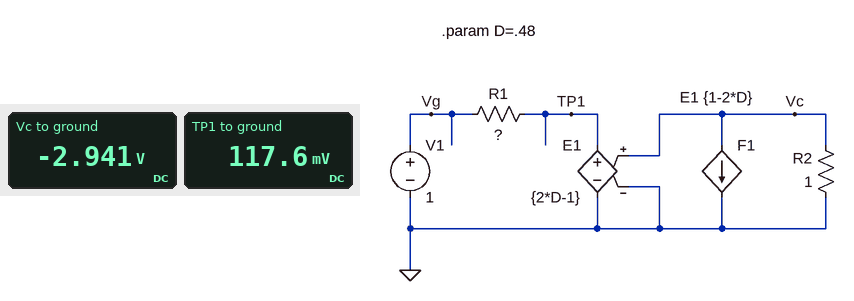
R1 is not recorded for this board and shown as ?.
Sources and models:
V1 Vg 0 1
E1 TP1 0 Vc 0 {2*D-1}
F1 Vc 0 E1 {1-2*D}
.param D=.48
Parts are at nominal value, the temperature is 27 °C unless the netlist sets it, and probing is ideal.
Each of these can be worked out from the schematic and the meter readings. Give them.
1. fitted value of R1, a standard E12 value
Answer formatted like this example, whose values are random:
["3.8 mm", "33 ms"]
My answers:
["0.012 Ω"]
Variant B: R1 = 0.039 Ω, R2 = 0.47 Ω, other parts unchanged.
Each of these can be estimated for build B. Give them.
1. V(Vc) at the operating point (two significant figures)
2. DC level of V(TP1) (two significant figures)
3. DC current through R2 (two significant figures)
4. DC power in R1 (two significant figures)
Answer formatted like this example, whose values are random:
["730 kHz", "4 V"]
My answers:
["-470 mV", "19 mV", "1.0 A", "25 W"]
